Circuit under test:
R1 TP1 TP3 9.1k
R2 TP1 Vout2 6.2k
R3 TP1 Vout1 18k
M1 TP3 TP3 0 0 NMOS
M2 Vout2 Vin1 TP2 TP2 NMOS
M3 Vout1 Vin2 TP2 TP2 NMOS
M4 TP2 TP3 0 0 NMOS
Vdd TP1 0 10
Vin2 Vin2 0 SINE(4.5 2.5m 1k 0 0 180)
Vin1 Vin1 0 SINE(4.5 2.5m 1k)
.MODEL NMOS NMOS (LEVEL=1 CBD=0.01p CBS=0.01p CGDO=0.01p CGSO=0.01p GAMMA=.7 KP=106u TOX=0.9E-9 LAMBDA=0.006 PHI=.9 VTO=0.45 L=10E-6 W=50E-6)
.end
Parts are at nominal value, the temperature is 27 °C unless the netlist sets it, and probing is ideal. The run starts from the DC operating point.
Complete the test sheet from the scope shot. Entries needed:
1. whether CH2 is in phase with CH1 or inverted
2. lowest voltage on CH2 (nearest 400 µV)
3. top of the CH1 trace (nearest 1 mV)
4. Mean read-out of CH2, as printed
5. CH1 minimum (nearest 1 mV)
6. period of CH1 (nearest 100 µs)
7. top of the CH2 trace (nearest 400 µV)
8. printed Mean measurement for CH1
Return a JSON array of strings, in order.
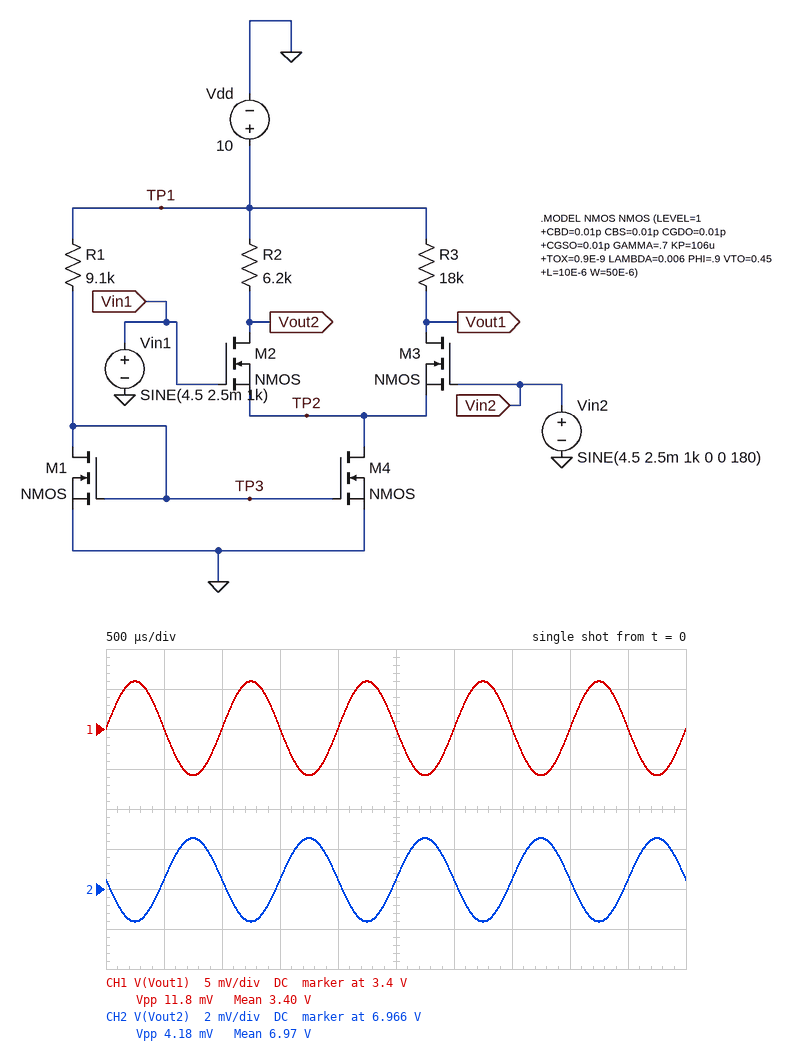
["inverted", "6.9644 V", "3.406 V", "6.97 V", "3.394 V", "1.0 ms", "6.9684 V", "3.40 V"]
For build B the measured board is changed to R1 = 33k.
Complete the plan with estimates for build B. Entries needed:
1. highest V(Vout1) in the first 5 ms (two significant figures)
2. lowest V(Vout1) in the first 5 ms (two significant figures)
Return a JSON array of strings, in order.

["7.7 V", "7.6 V"]
